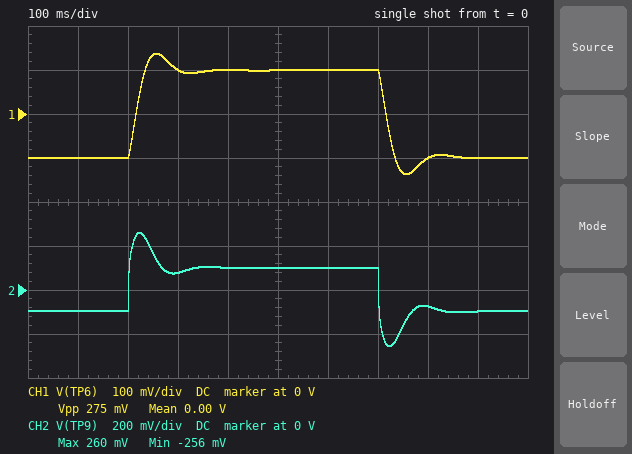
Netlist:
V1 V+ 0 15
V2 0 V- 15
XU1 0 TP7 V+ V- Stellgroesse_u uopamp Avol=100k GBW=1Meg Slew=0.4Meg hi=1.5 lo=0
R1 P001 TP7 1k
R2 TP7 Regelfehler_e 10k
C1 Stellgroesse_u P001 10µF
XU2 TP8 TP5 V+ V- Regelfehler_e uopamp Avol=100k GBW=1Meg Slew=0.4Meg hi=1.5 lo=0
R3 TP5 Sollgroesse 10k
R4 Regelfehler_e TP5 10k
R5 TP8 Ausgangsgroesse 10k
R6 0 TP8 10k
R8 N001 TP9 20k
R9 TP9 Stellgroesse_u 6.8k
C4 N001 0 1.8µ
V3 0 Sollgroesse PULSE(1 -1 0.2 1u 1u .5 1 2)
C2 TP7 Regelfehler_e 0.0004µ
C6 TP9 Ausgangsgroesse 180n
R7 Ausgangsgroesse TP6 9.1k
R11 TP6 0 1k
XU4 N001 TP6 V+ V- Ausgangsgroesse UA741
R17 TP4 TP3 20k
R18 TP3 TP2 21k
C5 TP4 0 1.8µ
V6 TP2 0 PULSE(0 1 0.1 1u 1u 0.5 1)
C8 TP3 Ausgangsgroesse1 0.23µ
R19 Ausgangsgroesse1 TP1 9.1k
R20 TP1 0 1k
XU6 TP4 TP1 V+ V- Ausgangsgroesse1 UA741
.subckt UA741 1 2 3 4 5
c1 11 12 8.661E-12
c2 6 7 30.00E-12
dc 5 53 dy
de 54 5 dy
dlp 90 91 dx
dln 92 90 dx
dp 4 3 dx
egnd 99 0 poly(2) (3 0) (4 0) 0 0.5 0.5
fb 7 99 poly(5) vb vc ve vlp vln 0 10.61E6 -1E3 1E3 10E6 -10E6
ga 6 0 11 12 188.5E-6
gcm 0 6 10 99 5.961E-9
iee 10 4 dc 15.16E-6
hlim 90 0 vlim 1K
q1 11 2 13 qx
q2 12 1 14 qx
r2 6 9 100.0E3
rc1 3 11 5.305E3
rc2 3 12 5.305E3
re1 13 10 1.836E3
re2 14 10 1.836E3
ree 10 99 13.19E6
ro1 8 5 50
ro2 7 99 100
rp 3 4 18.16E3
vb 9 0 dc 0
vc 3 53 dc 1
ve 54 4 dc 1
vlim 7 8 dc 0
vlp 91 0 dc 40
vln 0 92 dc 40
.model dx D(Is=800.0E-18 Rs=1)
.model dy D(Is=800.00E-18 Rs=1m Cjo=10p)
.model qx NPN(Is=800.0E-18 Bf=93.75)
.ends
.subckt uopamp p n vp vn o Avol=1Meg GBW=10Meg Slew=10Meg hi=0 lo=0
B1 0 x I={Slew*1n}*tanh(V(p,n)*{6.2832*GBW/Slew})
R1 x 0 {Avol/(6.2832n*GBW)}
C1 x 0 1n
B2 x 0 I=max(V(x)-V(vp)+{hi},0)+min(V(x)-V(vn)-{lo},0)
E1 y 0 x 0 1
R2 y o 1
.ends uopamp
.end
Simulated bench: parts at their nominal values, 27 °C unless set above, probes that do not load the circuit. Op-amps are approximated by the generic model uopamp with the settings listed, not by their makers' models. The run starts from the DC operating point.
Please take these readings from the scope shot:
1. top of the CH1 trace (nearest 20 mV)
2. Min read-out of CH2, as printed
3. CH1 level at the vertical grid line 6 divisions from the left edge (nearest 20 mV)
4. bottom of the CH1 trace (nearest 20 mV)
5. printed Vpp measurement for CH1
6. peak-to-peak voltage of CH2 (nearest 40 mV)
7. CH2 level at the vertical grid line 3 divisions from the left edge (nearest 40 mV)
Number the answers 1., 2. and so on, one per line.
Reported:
1. 140 mV
2. -256 mV
3. 100 mV
4. -140 mV
5. 275 mV
6. 520 mV
7. 80 mV
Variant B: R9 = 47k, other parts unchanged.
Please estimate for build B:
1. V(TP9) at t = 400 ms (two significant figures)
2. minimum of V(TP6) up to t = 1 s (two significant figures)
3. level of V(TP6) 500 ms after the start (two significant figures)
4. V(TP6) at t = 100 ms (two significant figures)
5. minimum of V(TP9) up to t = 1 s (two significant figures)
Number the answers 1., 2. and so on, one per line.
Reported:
1. 92 mV
2. -180 mV
3. 100 mV
4. -99 mV
5. -320 mV
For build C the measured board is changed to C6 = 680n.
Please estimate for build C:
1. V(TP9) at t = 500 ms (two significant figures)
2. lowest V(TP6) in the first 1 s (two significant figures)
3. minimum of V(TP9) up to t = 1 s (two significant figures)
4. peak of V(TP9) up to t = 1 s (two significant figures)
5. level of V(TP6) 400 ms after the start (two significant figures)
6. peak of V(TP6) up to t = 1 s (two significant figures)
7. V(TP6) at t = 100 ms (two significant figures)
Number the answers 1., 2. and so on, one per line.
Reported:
1. 2.7 V
2. -1.5 V
3. -7.3 V
4. 6.7 V
5. 450 mV
6. 1.5 V
7. -99 mV
